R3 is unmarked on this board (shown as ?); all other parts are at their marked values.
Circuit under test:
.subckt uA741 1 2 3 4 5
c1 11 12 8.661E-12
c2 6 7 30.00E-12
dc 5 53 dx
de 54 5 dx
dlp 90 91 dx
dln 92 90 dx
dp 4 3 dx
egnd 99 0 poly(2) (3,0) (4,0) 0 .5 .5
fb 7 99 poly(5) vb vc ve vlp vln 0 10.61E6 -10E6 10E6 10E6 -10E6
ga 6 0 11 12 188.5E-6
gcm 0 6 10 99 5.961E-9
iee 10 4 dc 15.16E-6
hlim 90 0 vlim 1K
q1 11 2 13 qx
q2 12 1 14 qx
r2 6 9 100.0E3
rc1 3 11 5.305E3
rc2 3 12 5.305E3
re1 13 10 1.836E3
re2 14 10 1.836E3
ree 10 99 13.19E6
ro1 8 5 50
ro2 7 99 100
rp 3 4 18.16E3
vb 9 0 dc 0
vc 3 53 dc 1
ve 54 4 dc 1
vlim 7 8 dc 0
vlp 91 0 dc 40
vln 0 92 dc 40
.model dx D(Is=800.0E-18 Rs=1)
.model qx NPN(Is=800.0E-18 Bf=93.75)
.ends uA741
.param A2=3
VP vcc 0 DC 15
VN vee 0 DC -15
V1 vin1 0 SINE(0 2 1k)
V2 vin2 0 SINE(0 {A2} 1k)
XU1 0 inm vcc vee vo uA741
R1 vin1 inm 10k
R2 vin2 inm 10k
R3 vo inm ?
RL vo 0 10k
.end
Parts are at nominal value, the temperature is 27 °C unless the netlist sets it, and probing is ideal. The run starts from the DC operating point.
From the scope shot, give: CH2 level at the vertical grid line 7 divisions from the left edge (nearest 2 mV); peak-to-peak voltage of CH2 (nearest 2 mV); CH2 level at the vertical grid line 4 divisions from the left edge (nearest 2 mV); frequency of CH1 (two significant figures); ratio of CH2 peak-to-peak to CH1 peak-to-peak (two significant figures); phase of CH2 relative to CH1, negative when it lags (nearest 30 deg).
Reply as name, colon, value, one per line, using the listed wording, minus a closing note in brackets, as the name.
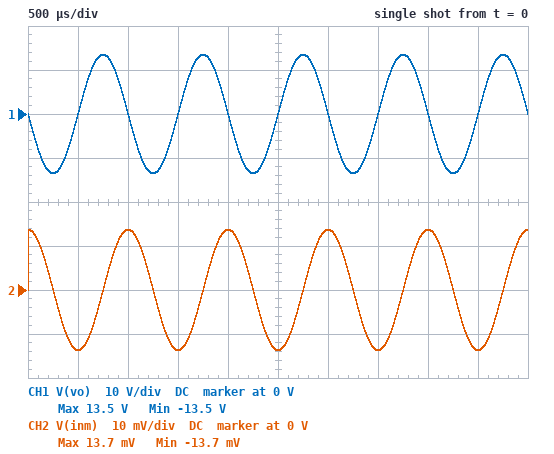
CH2 level at the vertical grid line 7 divisions from the left edge: -14 mV
peak-to-peak voltage of CH2: 28 mV
CH2 level at the vertical grid line 4 divisions from the left edge: 14 mV
frequency of CH1: 1.0 kHz
ratio of CH2 peak-to-peak to CH1 peak-to-peak: 0.0010
phase of CH2 relative to CH1, negative when it lags: -90 deg
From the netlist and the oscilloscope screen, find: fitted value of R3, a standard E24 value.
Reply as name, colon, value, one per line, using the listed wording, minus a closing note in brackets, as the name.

fitted value of R3, a standard E24 value: 27 kΩ
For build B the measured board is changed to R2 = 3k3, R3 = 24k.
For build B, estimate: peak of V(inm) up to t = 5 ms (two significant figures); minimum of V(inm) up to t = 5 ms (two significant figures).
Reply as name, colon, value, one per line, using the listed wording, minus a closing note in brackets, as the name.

peak of V(inm) up to t = 5 ms: 1.1 V
minimum of V(inm) up to t = 5 ms: -1.1 V
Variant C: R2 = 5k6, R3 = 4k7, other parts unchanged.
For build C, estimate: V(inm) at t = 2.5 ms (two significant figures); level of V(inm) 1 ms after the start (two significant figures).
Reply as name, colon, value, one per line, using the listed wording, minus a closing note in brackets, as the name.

V(inm) at t = 2.5 ms: -3.5 mV
level of V(inm) 1 ms after the start: 3.5 mV
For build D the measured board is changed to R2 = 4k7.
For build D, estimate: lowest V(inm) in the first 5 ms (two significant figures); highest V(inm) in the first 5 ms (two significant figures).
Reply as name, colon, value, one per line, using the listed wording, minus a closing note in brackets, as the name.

lowest V(inm) in the first 5 ms: -850 mV
highest V(inm) in the first 5 ms: 850 mV
